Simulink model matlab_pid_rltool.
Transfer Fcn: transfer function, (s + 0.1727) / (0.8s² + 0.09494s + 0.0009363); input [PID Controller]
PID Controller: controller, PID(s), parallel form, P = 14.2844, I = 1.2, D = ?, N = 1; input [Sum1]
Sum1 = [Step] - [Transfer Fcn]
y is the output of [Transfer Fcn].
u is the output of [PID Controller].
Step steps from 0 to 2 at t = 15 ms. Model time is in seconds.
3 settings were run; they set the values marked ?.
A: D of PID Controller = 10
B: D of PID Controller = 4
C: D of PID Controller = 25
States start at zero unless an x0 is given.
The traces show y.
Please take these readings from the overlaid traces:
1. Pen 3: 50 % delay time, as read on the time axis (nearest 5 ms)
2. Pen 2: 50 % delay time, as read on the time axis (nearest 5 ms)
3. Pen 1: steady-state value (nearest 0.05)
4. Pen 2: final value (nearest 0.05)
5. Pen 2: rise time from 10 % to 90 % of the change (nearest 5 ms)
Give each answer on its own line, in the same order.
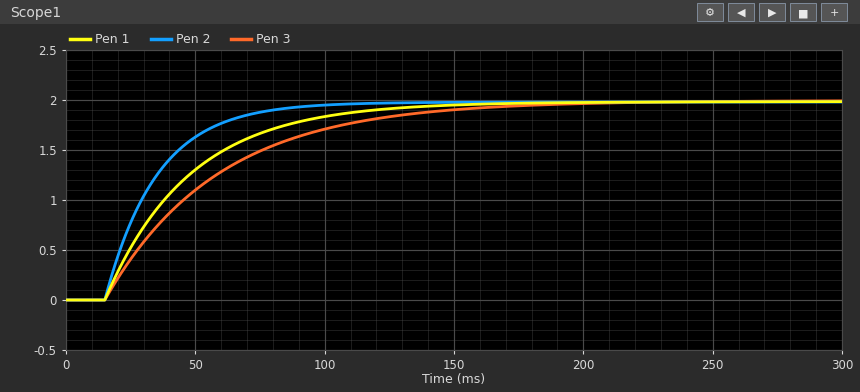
45 ms
30 ms
2.00
2.00
45 ms
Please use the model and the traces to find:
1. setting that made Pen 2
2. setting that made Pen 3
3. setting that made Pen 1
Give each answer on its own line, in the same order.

C
B
A
